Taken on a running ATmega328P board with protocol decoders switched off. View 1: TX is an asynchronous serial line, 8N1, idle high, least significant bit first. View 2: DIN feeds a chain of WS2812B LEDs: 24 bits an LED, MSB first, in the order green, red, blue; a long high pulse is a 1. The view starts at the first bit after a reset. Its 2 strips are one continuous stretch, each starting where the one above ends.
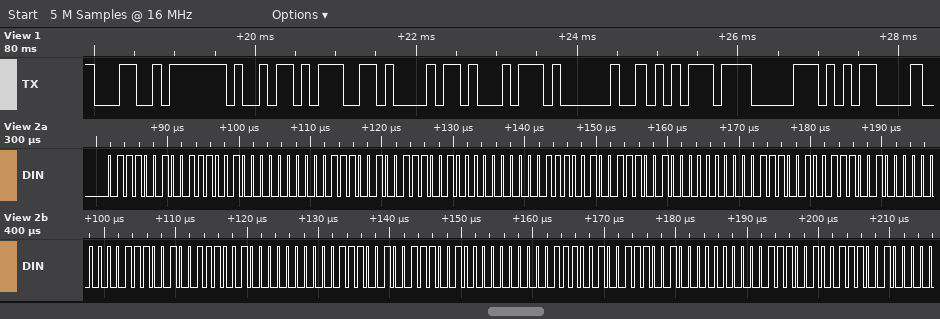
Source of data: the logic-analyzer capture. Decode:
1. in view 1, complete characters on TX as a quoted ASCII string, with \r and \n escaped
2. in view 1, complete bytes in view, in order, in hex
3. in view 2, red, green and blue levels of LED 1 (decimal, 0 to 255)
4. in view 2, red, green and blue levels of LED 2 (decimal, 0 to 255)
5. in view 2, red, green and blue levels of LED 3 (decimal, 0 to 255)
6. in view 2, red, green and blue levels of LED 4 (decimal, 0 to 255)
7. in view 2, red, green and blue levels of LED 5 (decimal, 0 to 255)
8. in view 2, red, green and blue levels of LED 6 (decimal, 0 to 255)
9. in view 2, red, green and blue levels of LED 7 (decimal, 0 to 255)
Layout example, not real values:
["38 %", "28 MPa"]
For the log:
["\"Light up\\r\"", "4C 69 67 68 74 20 75 70 0D", "114, 114, 0", "114, 114, 0", "114, 114, 0", "114, 114, 0", "114, 114, 0", "114, 114, 0", "114, 114, 0"]
